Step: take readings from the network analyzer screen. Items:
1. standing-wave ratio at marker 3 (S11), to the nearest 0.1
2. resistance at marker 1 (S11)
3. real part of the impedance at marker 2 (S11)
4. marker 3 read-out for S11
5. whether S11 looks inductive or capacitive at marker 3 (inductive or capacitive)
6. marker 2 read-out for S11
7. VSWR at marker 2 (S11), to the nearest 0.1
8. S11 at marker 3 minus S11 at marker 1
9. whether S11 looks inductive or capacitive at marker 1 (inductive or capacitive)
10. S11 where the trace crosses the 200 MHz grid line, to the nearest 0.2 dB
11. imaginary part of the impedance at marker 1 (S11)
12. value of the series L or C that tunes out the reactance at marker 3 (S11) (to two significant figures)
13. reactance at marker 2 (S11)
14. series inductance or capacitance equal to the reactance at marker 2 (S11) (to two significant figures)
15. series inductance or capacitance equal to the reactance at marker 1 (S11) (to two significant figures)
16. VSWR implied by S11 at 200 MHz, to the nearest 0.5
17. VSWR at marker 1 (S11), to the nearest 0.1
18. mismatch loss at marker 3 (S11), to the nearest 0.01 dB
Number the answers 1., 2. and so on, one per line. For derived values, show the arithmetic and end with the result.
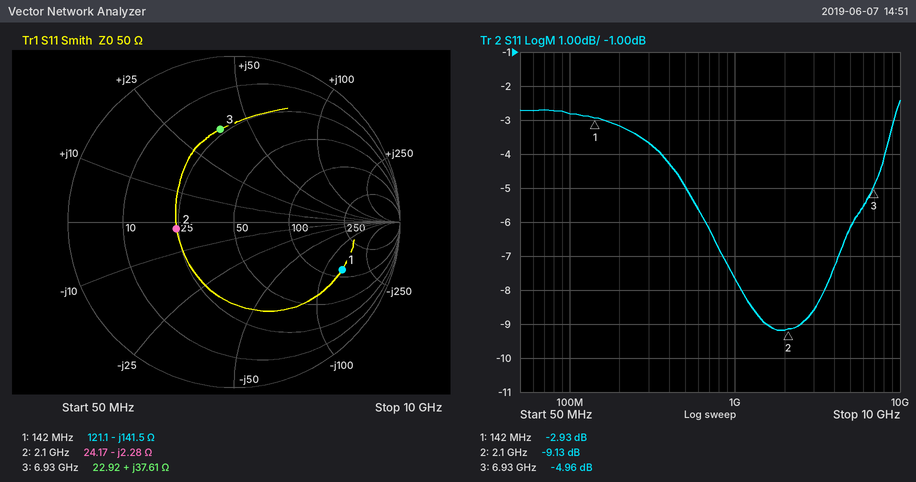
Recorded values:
1. 3.6
2. 121.1 Ω
3. 24.17 Ω
4. -4.96 dB
5. inductive
6. -9.13 dB
7. 2.1
8. -4.96 − (-2.93) = -2.03 dB
9. capacitive
10. -3.2 dB
11. -141.5 Ω
12. C = 1/(2π × 6.93 GHz × 37.61 Ω) ≈ 611 fF, so 610 fF to two significant figures
13. -2.28 Ω
14. C = 1/(2π × 2.1 GHz × 2.28 Ω) ≈ 33 pF
15. C = 1/(2π × 142 MHz × 141.5 Ω) ≈ 7.9 pF
16. |Γ| = 10^(-3.2/20) = 0.6918; VSWR = (1 + 0.6918)/(1 − 0.6918) ≈ 5.5
17. 6.0
18. −10 log10(1 − 10^(-4.96/10)) ≈ 1.67 dB
